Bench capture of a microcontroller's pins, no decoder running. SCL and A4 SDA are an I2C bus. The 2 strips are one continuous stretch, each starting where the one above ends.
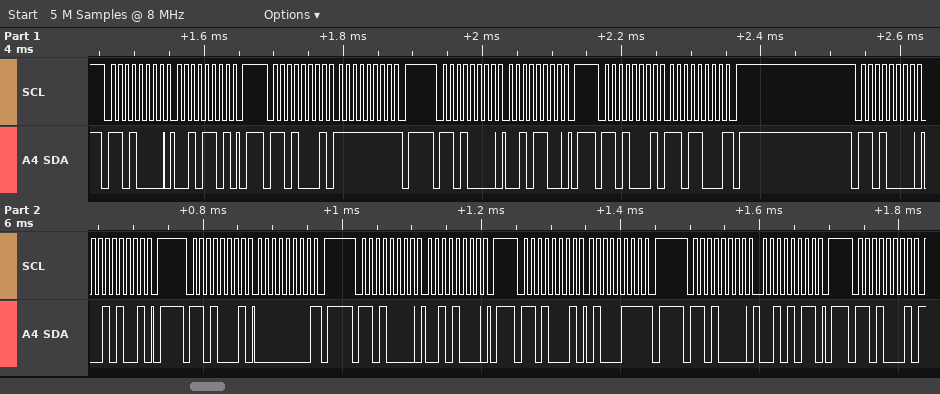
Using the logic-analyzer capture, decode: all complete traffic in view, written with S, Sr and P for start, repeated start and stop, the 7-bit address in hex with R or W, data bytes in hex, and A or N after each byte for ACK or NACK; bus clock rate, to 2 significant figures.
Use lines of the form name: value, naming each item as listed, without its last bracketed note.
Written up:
all complete traffic in view, written with S, Sr and P for start, repeated start and stop, the 7-bit address in hex with R or W, data bytes in hex, and A or N after each byte for ACK or NACK: S 68W A 2D A P S 68R A FF N P S 68W A 2C A P S 68R A D8 N P S 68W A 29 A P S 68R A 00 N P S 68W A 28 A P S 68R A 47 N P S 68W A 2B A P S 68R A
bus clock rate, to 2 significant figures: 100 kHz
